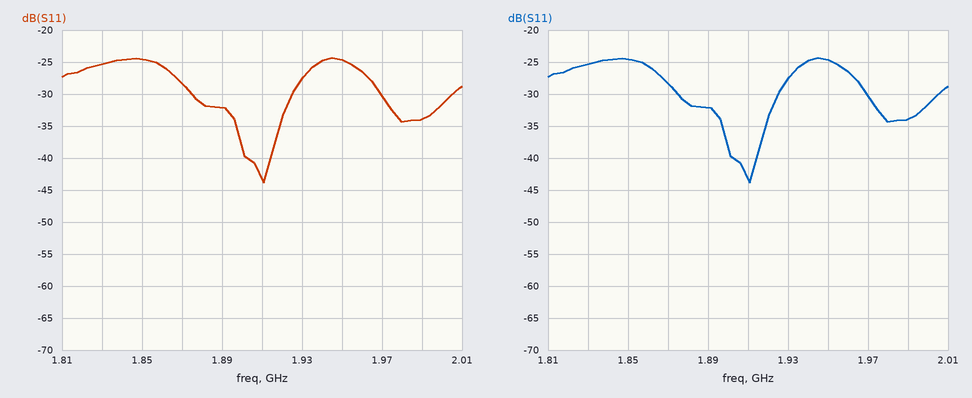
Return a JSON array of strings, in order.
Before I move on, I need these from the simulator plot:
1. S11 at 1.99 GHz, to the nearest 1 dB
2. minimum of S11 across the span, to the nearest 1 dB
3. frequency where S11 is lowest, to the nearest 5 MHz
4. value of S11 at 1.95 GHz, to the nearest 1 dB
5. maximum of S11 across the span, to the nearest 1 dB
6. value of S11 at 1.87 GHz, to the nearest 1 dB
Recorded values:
["-34 dB", "-44 dB", "1.910 GHz", "-25 dB", "-24 dB", "-28 dB"]
